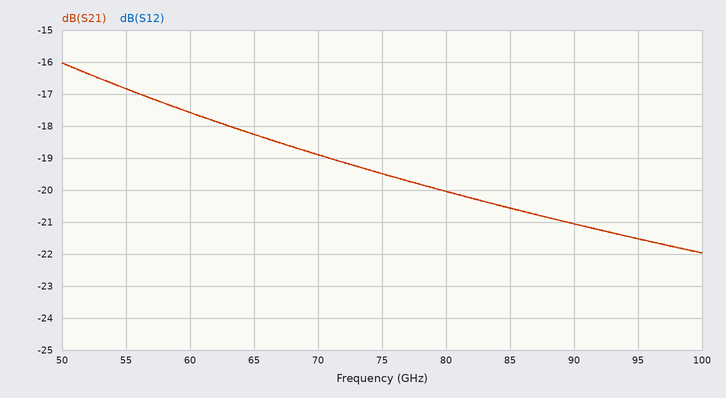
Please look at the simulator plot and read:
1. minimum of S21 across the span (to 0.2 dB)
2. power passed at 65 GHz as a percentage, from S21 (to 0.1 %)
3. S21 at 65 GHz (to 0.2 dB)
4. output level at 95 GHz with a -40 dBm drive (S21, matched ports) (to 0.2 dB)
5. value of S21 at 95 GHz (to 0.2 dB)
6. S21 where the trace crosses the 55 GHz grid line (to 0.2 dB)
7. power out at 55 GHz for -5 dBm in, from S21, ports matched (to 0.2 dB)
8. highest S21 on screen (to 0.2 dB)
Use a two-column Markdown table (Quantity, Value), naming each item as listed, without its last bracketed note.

| Quantity | Value |
|---|---|
| minimum of S21 across the span | -22.0 dB |
| power passed at 65 GHz as a percentage, from S21 | 1.5 % |
| S21 at 65 GHz | -18.2 dB |
| output level at 95 GHz with a -40 dBm drive (S21, matched ports) | -61.6 dBm |
| value of S21 at 95 GHz | -21.6 dB |
| S21 where the trace crosses the 55 GHz grid line | -16.8 dB |
| power out at 55 GHz for -5 dBm in, from S21, ports matched | -21.8 dBm |
| highest S21 on screen | -16.0 dB |
